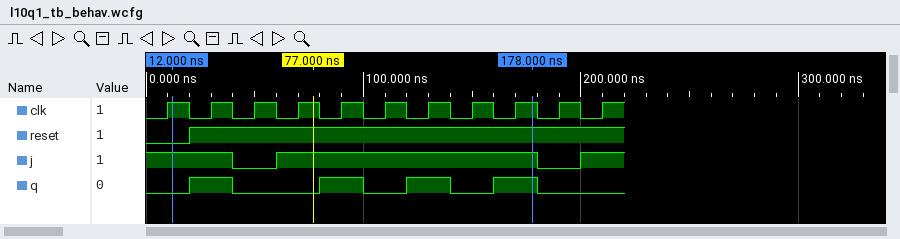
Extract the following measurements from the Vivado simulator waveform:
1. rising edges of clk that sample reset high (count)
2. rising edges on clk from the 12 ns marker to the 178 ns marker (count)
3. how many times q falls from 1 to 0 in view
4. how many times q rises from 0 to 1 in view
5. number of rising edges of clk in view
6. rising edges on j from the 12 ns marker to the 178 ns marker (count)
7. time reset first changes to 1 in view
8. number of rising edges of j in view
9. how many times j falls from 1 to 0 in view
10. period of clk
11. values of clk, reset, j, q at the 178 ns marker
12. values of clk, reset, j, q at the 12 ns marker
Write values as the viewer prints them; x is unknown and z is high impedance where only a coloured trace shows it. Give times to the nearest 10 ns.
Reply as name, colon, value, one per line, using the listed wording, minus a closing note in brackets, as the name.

rising edges of clk that sample reset high: 10
rising edges on clk from the 12 ns marker to the 178 ns marker: 8
how many times q falls from 1 to 0 in view: 4
how many times q rises from 0 to 1 in view: 4
number of rising edges of clk in view: 11
rising edges on j from the 12 ns marker to the 178 ns marker: 1
time reset first changes to 1 in view: 20 ns
number of rising edges of j in view: 2
how many times j falls from 1 to 0 in view: 2
period of clk: 20 ns
values of clk, reset, j, q at the 178 ns marker: clk=1, reset=1, j=1, q=1
values of clk, reset, j, q at the 12 ns marker: clk=1, reset=0, j=1, q=0
